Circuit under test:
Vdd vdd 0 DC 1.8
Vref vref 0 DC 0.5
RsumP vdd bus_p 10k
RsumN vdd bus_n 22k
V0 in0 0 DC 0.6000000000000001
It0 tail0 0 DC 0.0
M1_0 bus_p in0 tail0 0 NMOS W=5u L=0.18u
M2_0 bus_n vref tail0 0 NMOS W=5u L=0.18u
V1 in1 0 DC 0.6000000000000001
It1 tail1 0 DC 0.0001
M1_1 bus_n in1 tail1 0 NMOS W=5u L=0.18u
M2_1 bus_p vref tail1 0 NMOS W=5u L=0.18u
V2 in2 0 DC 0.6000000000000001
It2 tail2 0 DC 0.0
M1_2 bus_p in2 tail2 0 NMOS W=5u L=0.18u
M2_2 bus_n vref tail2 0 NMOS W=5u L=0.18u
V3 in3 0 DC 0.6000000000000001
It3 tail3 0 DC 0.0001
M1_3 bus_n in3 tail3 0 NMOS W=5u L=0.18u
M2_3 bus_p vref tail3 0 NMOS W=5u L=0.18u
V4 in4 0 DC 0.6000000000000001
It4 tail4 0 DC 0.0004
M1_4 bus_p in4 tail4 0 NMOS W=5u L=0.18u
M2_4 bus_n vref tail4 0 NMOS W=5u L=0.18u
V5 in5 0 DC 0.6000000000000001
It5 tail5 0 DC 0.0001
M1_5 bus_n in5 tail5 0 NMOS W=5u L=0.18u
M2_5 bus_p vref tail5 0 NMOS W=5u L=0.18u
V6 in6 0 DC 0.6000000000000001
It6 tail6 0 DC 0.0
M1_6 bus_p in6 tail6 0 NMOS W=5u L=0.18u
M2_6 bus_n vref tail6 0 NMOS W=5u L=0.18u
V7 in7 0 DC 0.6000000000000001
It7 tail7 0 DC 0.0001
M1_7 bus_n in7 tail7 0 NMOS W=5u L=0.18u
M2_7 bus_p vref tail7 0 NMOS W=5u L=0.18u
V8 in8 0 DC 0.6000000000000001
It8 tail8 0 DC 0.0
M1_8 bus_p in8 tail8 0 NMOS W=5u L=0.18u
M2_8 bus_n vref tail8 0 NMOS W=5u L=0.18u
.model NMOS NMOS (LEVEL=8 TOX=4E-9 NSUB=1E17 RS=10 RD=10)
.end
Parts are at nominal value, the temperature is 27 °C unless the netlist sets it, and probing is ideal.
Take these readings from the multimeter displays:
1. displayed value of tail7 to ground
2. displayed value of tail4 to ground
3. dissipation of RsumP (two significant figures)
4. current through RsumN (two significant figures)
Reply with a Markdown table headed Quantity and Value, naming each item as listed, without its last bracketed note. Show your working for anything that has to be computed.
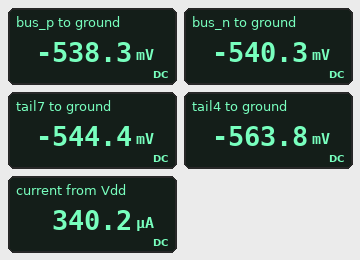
| Quantity | Value |
|---|---|
| displayed value of tail7 to ground | -544.4 mV |
| displayed value of tail4 to ground | -563.8 mV |
| dissipation of RsumP | (1.8 V - (-538.3 mV))^2 / 10 kΩ = 550 µW |
| current through RsumN | (1.8 V - (-540.3 mV)) / 22 kΩ = 110 µA |
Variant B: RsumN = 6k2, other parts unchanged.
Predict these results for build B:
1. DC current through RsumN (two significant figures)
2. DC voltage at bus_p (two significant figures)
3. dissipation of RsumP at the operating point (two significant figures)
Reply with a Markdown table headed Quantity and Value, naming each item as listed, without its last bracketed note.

| Quantity | Value |
|---|---|
| DC current through RsumN | 370 µA |
| DC voltage at bus_p | -520 mV |
| dissipation of RsumP at the operating point | 540 µW |
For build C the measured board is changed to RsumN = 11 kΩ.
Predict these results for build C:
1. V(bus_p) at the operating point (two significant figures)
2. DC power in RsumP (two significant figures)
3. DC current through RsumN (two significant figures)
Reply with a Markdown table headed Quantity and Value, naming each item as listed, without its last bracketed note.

| Quantity | Value |
|---|---|
| V(bus_p) at the operating point | -530 mV |
| DC power in RsumP | 540 µW |
| DC current through RsumN | 210 µA |
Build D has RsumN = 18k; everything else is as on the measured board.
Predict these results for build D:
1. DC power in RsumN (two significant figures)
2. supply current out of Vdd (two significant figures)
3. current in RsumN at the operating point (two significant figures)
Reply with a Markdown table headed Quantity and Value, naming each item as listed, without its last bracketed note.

| Quantity | Value |
|---|---|
| DC power in RsumN | 300 µW |
| supply current out of Vdd | 360 µA |
| current in RsumN at the operating point | 130 µA |
